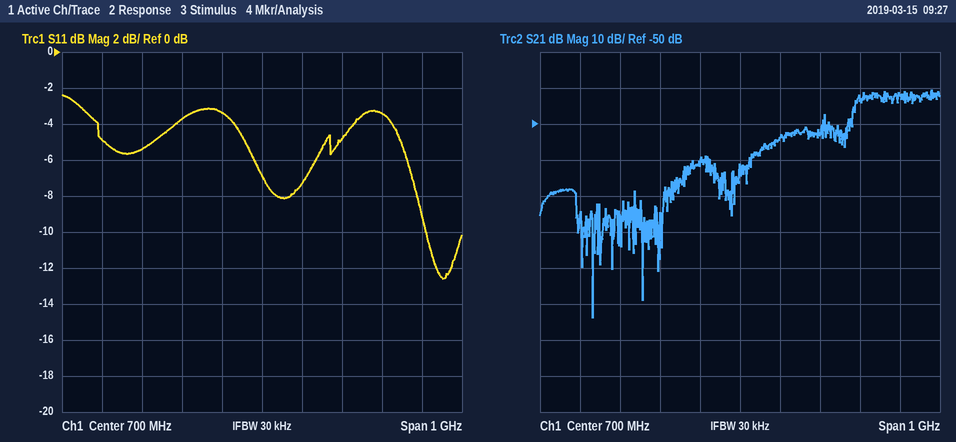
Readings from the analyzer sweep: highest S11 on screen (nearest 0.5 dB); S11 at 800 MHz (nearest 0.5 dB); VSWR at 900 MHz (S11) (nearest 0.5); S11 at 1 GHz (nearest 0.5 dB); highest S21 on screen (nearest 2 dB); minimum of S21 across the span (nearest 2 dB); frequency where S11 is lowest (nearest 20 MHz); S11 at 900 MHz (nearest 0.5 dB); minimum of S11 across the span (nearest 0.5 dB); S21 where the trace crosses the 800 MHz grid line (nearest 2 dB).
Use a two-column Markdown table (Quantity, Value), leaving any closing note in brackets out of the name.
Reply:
| Quantity | Value |
|---|---|
| highest S11 on screen | -2.5 dB |
| S11 at 800 MHz | -7.5 dB |
| VSWR at 900 MHz (S11) | 3.5 |
| S11 at 1 GHz | -3.5 dB |
| highest S21 on screen | -40 dB |
| minimum of S21 across the span | -104 dB |
| frequency where S11 is lowest | 1.16 GHz |
| S11 at 900 MHz | -5.0 dB |
| minimum of S11 across the span | -12.5 dB |
| S21 where the trace crosses the 800 MHz grid line | -54 dB |
